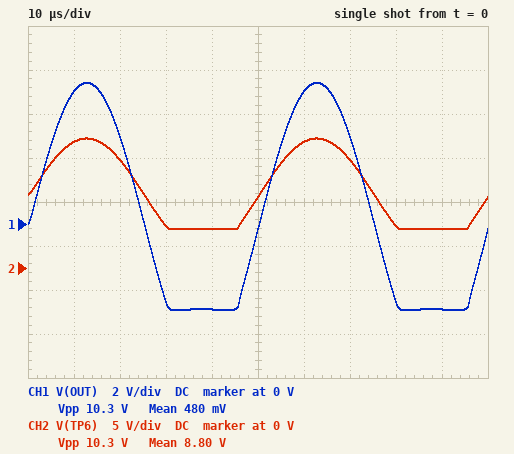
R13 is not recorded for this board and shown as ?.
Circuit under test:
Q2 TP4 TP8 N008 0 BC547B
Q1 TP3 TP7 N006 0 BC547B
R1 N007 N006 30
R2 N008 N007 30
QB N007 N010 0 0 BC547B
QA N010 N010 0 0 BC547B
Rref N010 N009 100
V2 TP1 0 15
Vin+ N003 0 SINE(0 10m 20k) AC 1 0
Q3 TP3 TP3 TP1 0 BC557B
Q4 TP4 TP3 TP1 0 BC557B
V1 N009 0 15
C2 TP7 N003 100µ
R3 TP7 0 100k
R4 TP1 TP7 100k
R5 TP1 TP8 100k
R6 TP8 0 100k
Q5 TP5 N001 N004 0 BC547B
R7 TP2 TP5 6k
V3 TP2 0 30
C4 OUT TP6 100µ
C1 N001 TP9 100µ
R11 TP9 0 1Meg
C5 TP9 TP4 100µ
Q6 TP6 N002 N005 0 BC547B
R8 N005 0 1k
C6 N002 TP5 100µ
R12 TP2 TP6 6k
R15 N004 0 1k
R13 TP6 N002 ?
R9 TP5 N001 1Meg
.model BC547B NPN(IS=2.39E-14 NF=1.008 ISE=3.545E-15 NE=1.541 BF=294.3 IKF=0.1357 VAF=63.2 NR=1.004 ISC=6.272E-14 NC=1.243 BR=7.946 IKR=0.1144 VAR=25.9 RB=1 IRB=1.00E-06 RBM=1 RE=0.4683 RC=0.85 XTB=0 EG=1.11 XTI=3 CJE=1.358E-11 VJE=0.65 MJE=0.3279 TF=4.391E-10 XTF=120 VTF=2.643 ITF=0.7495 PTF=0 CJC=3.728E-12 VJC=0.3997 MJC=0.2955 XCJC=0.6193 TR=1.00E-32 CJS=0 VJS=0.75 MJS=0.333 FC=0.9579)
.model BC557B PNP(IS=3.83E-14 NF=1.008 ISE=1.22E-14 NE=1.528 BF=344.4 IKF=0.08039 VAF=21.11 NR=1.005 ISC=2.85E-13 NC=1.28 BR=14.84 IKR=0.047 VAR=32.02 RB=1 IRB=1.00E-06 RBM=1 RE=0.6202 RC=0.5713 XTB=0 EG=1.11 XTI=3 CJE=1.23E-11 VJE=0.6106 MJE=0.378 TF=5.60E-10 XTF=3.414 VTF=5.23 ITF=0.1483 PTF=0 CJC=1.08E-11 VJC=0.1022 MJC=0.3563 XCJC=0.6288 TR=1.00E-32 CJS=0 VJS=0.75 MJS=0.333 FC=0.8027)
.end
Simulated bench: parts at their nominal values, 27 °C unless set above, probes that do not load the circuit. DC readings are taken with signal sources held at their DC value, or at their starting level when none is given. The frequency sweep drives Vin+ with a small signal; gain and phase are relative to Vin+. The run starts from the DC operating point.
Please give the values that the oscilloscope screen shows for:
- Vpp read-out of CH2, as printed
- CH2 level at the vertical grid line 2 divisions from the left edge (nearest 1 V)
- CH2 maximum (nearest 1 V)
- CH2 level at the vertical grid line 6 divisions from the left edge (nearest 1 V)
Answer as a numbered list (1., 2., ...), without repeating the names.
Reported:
1. 10.3 V
2. 12 V
3. 15 V
4. 14 V
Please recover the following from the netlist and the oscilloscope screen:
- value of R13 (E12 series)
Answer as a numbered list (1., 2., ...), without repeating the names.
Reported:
1. 330 kΩ
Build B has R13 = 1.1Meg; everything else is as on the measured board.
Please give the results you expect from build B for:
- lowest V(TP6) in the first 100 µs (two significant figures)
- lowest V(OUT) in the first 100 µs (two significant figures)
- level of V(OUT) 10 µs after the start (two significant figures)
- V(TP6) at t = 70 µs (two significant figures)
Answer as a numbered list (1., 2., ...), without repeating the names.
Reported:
1. 6.0 V
2. -7.1 V
3. 6.6 V
4. 17 V
